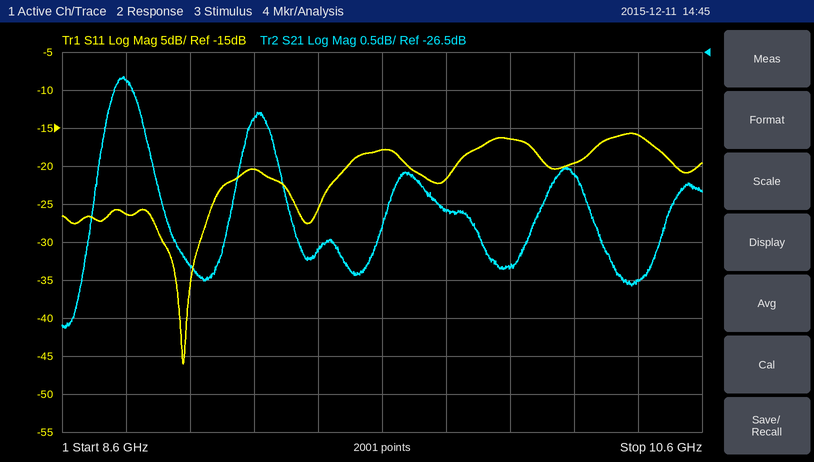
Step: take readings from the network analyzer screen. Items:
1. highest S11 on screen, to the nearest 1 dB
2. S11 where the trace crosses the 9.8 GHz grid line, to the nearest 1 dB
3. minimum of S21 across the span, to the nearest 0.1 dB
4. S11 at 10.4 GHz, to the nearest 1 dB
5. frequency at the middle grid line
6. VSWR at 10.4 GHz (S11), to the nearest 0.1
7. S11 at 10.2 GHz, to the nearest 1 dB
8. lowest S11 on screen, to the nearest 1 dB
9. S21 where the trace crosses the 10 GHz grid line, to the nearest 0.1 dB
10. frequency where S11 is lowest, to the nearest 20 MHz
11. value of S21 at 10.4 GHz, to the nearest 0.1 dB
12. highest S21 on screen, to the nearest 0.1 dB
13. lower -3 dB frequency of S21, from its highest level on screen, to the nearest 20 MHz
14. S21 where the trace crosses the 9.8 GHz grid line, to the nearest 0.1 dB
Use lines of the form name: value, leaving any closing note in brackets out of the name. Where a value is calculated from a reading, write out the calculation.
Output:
highest S11 on screen, to the nearest 1 dB: -16 dB
S11 where the trace crosses the 9.8 GHz grid line, to the nearest 1 dB: -22 dB
minimum of S21 across the span, to the nearest 0.1 dB: -30.1 dB
S11 at 10.4 GHz, to the nearest 1 dB: -16 dB
frequency at the middle grid line: 9.6 GHz
VSWR at 10.4 GHz (S11), to the nearest 0.1: |Γ| = 10^(-16/20) = 0.1585; VSWR = (1 + 0.1585)/(1 − 0.1585) ≈ 1.4
S11 at 10.2 GHz, to the nearest 1 dB: -20 dB
lowest S11 on screen, to the nearest 1 dB: -46 dB
S21 where the trace crosses the 10 GHz grid line, to the nearest 0.1 dB: -29.3 dB
frequency where S11 is lowest, to the nearest 20 MHz: 8.98 GHz
value of S21 at 10.4 GHz, to the nearest 0.1 dB: -29.5 dB
highest S21 on screen, to the nearest 0.1 dB: -26.8 dB
lower -3 dB frequency of S21, from its highest level on screen, to the nearest 20 MHz: 8.64 GHz
S21 where the trace crosses the 9.8 GHz grid line, to the nearest 0.1 dB: -28.6 dB
